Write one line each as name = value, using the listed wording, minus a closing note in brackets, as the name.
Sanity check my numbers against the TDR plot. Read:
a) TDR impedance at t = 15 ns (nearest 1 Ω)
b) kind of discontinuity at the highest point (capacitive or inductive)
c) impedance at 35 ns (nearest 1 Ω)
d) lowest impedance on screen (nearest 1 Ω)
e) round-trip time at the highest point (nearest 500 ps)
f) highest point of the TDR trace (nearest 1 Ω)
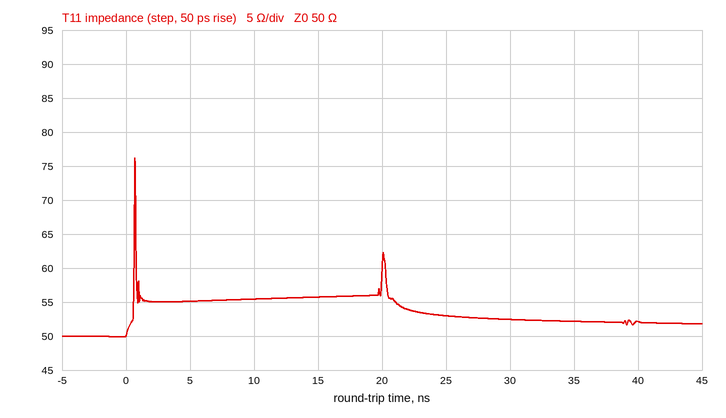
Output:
TDR impedance at t = 15 ns = 56 Ω
kind of discontinuity at the highest point = inductive
impedance at 35 ns = 52 Ω
lowest impedance on screen = 50 Ω
round-trip time at the highest point = 500 ps
highest point of the TDR trace = 76 Ω
